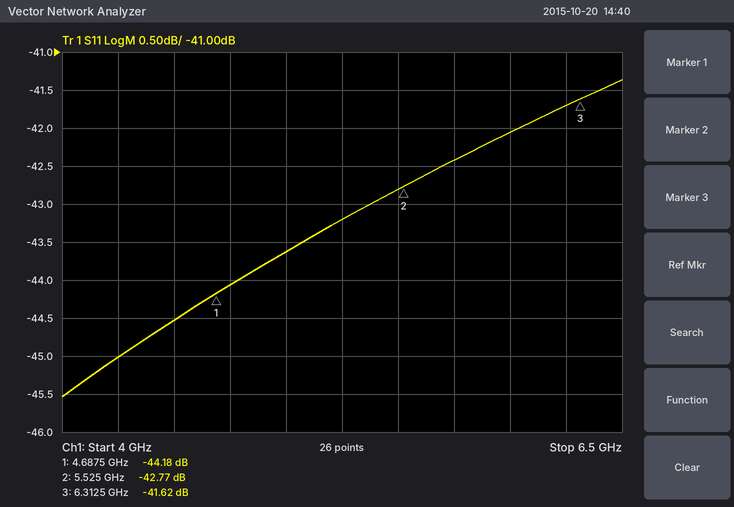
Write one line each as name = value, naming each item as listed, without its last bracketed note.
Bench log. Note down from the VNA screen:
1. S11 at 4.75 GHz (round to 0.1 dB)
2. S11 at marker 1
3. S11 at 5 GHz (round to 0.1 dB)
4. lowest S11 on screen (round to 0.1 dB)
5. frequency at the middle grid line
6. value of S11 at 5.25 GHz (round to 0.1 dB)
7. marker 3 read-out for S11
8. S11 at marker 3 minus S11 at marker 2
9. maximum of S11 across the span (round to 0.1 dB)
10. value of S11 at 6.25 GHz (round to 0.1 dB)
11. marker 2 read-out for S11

S11 at 4.75 GHz = -44.1 dB
S11 at marker 1 = -44.18 dB
S11 at 5 GHz = -43.6 dB
lowest S11 on screen = -45.5 dB
frequency at the middle grid line = 5.25 GHz
value of S11 at 5.25 GHz = -43.2 dB
marker 3 read-out for S11 = -41.62 dB
S11 at marker 3 minus S11 at marker 2 = 1.15 dB
maximum of S11 across the span = -41.4 dB
value of S11 at 6.25 GHz = -41.7 dB
marker 2 read-out for S11 = -42.77 dB
